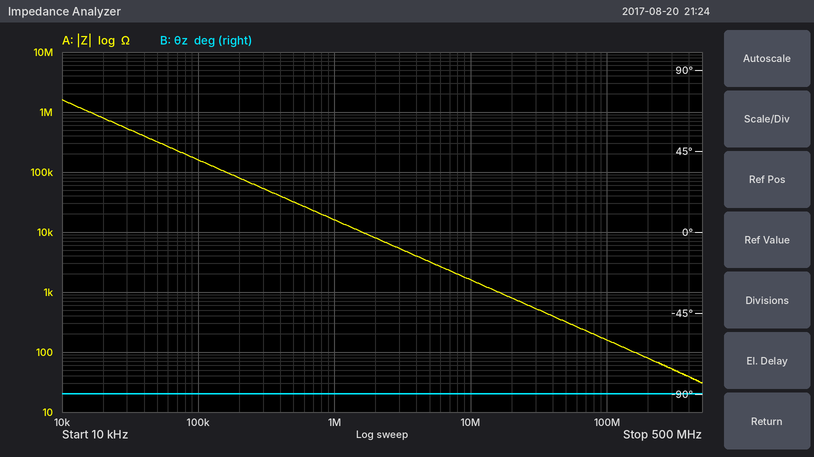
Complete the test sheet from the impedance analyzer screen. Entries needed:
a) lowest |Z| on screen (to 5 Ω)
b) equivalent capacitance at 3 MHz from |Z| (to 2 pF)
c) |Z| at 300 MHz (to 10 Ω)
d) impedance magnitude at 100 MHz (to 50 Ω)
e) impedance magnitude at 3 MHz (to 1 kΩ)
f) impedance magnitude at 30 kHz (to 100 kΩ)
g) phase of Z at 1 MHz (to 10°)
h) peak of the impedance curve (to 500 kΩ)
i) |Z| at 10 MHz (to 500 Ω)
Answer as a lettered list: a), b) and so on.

a) 30 Ω
b) 10 pF
c) 50 Ω
d) 150 Ω
e) 5 kΩ
f) 500 kΩ
g) -90°
h) 1.5 MΩ
i) 1.5 kΩ
